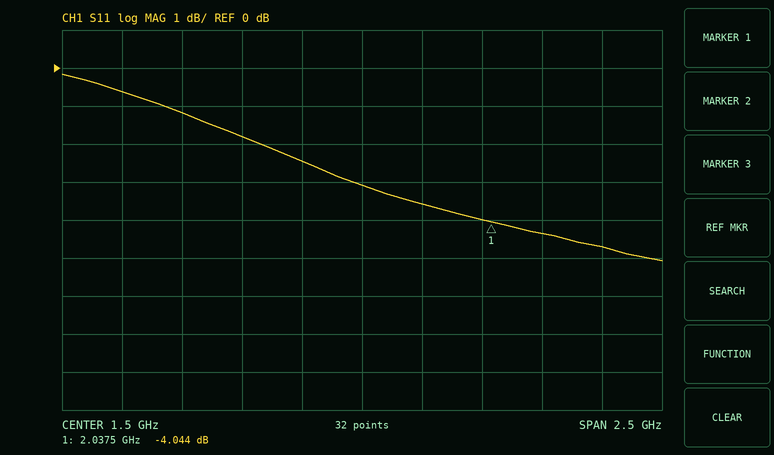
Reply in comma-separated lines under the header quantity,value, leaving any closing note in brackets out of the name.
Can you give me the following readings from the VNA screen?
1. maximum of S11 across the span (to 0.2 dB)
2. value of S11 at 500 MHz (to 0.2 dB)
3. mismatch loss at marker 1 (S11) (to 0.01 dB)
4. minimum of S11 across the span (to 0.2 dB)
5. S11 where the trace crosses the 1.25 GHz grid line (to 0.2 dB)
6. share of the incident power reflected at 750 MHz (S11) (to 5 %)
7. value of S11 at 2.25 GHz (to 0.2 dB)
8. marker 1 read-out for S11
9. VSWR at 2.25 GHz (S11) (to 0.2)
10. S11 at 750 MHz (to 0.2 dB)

quantity,value
maximum of S11 across the span,-0.2 dB
value of S11 at 500 MHz,-0.6 dB
mismatch loss at marker 1 (S11),2.18 dB
minimum of S11 across the span,-5.0 dB
S11 where the trace crosses the 1.25 GHz grid line,-2.4 dB
share of the incident power reflected at 750 MHz (S11),75 %
value of S11 at 2.25 GHz,-4.4 dB
marker 1 read-out for S11,-4.044 dB
VSWR at 2.25 GHz (S11),4.0
S11 at 750 MHz,-1.2 dB
